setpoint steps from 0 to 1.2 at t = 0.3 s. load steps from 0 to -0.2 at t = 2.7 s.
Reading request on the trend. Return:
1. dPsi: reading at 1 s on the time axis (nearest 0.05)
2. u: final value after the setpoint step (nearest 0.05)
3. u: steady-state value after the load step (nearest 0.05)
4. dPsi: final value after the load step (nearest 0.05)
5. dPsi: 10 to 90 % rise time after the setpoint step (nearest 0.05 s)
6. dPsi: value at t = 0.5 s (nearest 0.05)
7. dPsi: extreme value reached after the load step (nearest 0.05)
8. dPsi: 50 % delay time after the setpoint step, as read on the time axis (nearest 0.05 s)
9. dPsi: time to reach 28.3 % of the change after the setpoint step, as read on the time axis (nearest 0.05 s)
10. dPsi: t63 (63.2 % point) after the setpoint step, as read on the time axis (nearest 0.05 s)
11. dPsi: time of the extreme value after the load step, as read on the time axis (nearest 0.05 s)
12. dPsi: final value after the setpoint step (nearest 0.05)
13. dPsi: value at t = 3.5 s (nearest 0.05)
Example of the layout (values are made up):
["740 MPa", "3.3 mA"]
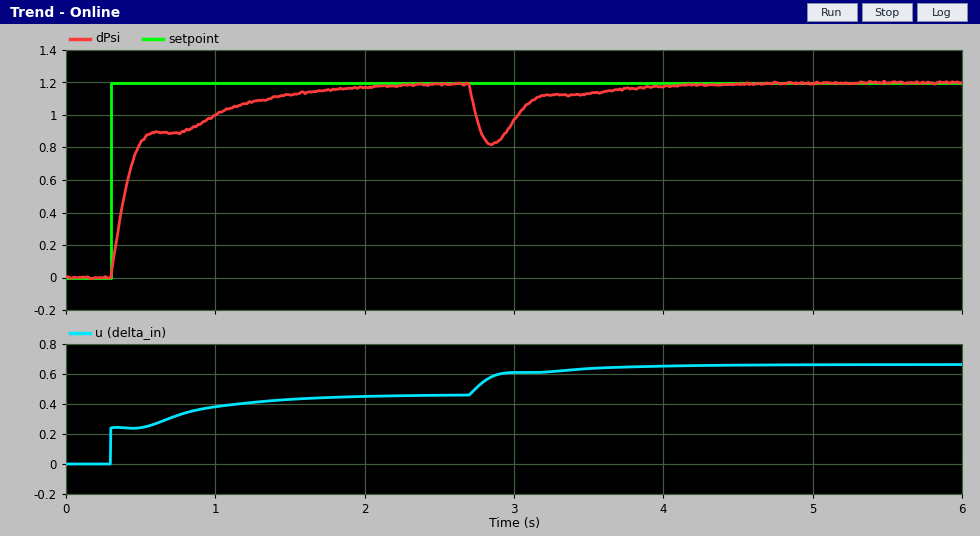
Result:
["1.00", "0.45", "0.65", "1.20", "0.90 s", "0.85", "0.80", "0.40 s", "0.35 s", "0.45 s", "2.85 s", "1.20", "1.15"]
